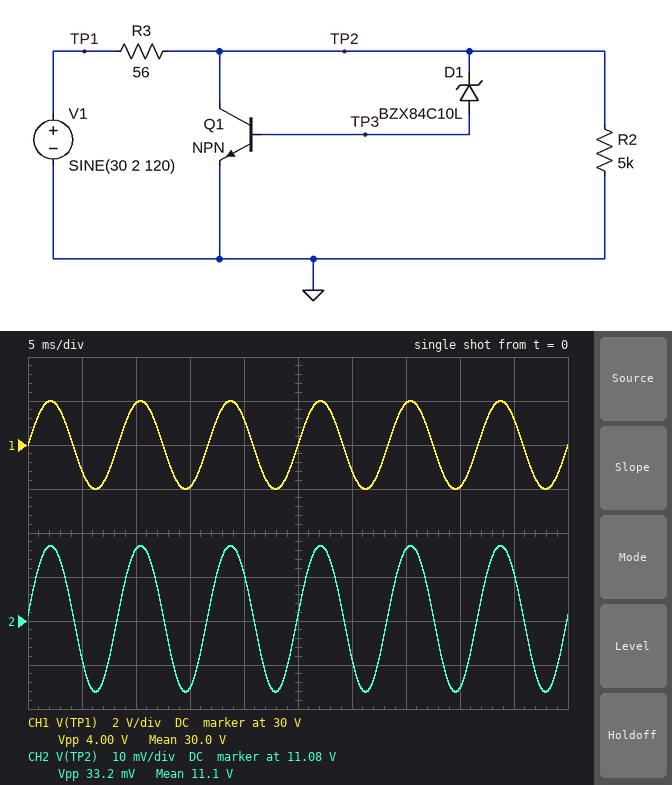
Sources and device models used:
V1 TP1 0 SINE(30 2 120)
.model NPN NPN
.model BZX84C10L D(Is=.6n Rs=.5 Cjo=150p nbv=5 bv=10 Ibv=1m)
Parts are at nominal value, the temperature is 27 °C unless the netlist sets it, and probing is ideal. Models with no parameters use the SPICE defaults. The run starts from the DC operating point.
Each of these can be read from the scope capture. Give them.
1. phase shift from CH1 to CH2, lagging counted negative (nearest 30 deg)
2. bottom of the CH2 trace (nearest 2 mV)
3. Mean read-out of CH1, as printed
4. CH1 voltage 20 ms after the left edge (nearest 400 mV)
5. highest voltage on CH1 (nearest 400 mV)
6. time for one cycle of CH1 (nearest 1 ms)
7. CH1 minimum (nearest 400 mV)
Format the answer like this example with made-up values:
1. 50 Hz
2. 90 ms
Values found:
1. 0 deg
2. 11.064 V
3. 30.0 V
4. 31.2 V
5. 32.0 V
6. 8 ms
7. 28.0 V
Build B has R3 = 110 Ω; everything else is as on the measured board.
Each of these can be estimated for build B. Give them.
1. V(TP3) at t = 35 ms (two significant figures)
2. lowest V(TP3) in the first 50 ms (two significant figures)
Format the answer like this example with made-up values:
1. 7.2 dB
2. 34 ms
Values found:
1. 910 mV
2. 900 mV
